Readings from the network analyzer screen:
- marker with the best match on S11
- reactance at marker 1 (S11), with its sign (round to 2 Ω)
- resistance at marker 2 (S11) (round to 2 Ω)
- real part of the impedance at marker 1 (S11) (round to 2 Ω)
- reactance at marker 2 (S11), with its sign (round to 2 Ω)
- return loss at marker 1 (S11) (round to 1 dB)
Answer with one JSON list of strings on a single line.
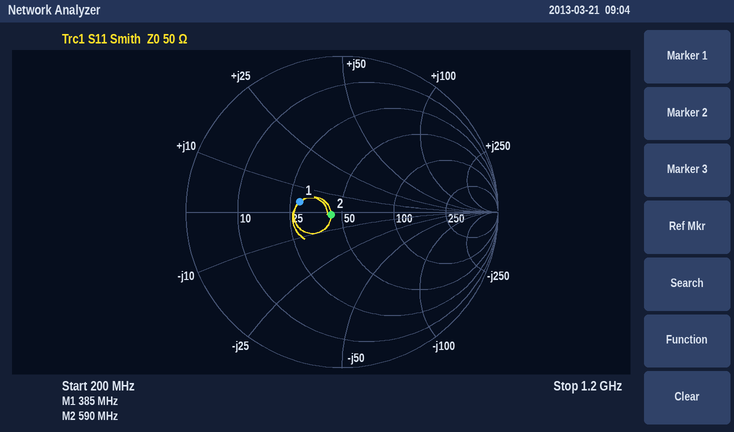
["marker 2", "+4 Ω", "44 Ω", "28 Ω", "-2 Ω", "11 dB"]
